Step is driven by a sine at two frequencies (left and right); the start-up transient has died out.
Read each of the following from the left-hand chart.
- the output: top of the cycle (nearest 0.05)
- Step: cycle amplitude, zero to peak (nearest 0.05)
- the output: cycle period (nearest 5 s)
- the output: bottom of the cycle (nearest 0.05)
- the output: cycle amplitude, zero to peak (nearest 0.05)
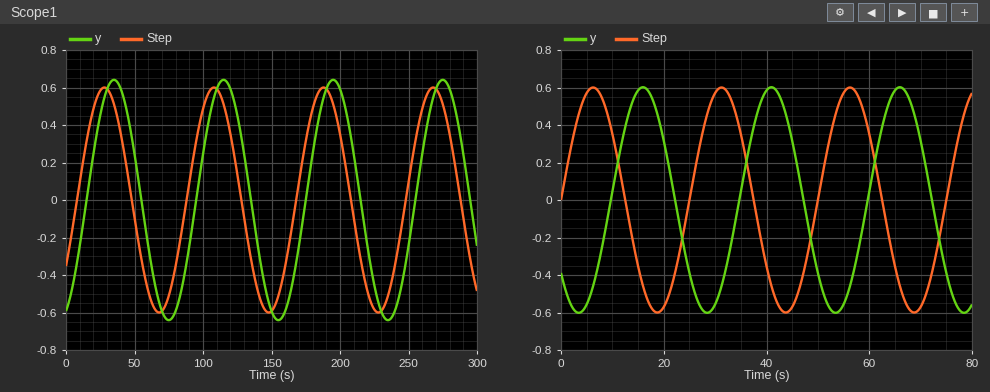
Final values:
0.65
0.60
80 s
-0.65
0.65
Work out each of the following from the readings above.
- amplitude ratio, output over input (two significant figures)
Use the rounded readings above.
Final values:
1.1
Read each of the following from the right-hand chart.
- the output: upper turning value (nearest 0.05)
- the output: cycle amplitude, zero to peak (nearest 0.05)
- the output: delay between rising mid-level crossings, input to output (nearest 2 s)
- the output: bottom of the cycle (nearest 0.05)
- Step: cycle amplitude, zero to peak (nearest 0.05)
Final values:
0.60
0.60
10 s
-0.60
0.60
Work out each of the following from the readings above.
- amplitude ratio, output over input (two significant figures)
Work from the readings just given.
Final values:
1.0
